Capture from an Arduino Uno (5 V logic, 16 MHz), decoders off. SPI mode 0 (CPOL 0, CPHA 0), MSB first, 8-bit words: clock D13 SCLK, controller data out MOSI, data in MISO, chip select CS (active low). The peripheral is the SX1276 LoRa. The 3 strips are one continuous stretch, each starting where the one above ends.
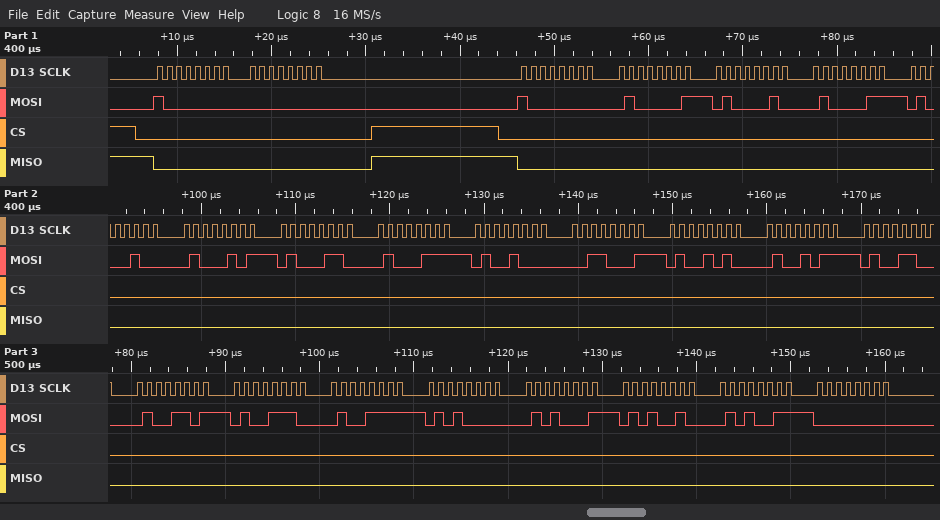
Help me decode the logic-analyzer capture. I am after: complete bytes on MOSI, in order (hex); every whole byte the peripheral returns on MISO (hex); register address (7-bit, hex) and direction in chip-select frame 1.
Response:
80 00 80 41 42 43 44 45 46 47 48 31 4A 4B 4C 4D 4E 4F 50 51 52 53 00
00 00 00 00 00 00 00 00 00 00 00 00 00 00 00 00 00 00 00 00 00 00 00
0x00 write
